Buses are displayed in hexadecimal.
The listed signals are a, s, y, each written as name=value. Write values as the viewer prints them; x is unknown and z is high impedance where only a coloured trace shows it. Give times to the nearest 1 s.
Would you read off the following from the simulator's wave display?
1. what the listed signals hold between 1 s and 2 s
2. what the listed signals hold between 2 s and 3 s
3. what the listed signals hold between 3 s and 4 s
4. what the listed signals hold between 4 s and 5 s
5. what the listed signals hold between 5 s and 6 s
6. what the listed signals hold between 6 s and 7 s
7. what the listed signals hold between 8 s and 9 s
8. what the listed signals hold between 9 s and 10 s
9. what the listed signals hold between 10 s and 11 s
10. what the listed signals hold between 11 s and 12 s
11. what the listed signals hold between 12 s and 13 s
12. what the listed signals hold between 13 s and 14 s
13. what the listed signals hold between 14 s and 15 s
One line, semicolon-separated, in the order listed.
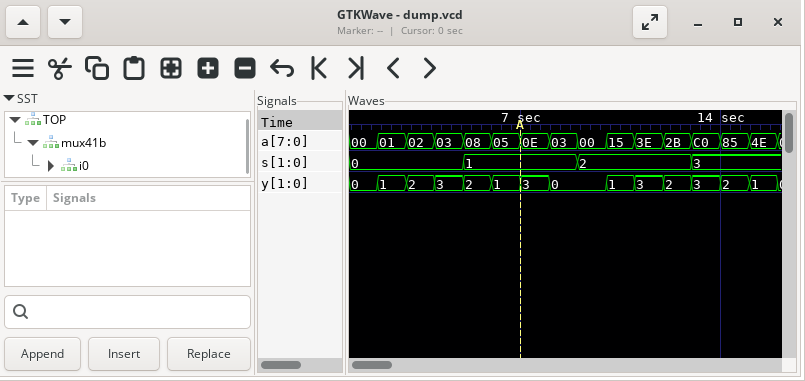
a=00, s=0, y=0; a=01, s=0, y=1; a=02, s=0, y=2; a=03, s=0, y=3; a=08, s=1, y=2; a=05, s=1, y=1; a=03, s=1, y=0; a=00, s=2, y=0; a=15, s=2, y=1; a=3E, s=2, y=3; a=2B, s=2, y=2; a=C0, s=3, y=3; a=85, s=3, y=2
